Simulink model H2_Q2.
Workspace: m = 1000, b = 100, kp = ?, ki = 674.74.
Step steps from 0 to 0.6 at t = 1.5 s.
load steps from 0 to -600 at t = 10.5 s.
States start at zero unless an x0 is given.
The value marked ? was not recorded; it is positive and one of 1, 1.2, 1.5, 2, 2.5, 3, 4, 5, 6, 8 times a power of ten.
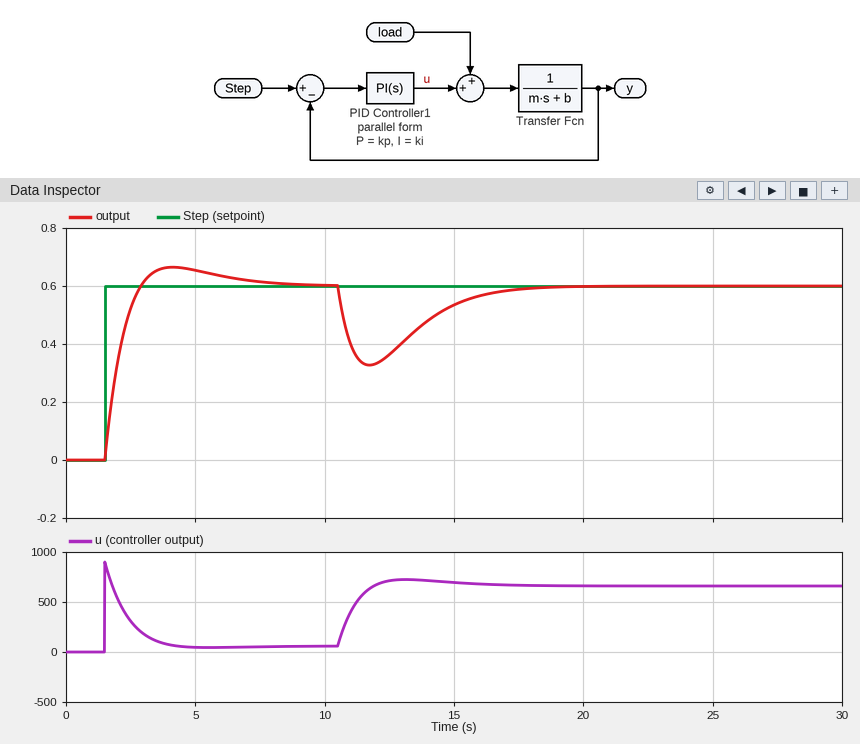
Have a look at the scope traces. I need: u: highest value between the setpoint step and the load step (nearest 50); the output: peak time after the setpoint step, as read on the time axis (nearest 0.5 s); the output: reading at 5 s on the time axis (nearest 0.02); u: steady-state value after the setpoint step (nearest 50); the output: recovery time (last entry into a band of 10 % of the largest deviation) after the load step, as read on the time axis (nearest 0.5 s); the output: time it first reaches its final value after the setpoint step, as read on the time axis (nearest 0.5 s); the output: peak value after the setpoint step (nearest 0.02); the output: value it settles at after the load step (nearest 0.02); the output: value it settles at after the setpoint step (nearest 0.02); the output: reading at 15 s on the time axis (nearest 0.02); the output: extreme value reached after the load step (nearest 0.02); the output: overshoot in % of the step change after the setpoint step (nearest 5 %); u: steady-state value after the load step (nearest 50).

900
4.0 s
0.66
50
16.5 s
3.0 s
0.66
0.60
0.60
0.54
0.32
10 %
650
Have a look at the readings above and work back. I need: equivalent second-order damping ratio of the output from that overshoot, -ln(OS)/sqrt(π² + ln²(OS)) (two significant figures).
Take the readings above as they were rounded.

0.59
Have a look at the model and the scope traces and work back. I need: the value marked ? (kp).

1500
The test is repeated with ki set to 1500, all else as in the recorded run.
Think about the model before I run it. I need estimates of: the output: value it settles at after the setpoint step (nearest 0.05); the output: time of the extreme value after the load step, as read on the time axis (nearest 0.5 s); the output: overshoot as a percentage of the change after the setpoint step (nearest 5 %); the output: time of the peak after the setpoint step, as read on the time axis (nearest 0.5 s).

0.60
11.5 s
20 %
3.5 s
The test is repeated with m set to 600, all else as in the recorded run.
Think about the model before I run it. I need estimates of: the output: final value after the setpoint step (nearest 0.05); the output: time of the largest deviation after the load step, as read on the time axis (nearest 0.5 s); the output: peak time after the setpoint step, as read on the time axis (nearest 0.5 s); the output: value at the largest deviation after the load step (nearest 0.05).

0.60
11.5 s
3.5 s
0.30
